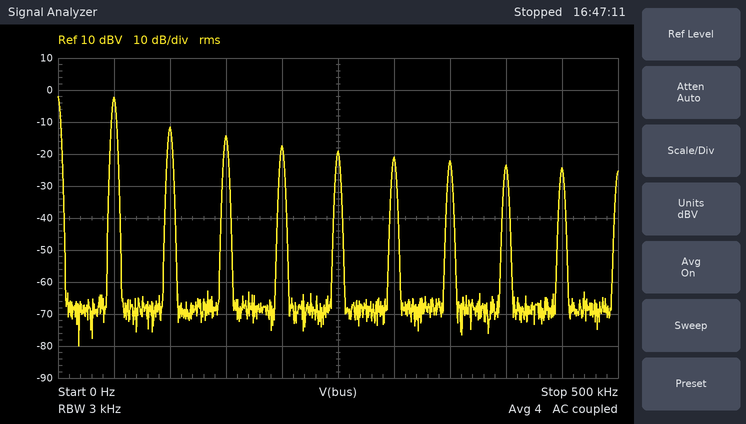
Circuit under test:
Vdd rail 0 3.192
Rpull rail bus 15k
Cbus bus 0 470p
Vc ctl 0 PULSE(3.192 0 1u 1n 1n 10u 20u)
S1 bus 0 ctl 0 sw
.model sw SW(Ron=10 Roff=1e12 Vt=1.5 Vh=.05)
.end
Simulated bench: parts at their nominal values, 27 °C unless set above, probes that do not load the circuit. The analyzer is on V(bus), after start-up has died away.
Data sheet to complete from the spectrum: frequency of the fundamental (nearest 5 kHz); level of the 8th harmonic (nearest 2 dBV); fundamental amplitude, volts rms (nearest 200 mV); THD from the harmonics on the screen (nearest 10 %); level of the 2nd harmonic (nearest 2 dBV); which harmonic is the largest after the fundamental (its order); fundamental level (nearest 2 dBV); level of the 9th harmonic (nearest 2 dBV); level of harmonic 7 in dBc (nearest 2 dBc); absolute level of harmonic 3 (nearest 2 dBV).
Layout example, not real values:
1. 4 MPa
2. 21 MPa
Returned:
1. 50 kHz
2. -24 dBV
3. 800 mV
4. 50 %
5. -12 dBV
6. 2
7. -2 dBV
8. -24 dBV
9. -20 dBc
10. -14 dBV
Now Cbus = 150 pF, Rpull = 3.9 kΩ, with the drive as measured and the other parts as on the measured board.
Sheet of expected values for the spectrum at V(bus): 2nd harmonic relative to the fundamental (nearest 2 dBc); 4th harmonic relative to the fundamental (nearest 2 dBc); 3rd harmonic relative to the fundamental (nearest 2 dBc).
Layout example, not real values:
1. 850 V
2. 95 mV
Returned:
1. -22 dBc
2. -22 dBc
3. -10 dBc
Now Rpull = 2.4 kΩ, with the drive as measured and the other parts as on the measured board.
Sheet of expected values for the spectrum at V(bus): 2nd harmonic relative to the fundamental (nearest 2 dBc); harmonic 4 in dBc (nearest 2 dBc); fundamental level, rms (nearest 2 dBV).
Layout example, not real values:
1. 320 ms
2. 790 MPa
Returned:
1. -16 dBc
2. -20 dBc
3. 2 dBV
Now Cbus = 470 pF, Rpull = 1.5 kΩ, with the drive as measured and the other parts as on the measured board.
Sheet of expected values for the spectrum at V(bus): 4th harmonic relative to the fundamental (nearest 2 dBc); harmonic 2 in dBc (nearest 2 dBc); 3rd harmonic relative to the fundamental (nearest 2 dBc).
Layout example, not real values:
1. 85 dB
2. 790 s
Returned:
1. -22 dBc
2. -20 dBc
3. -10 dBc
